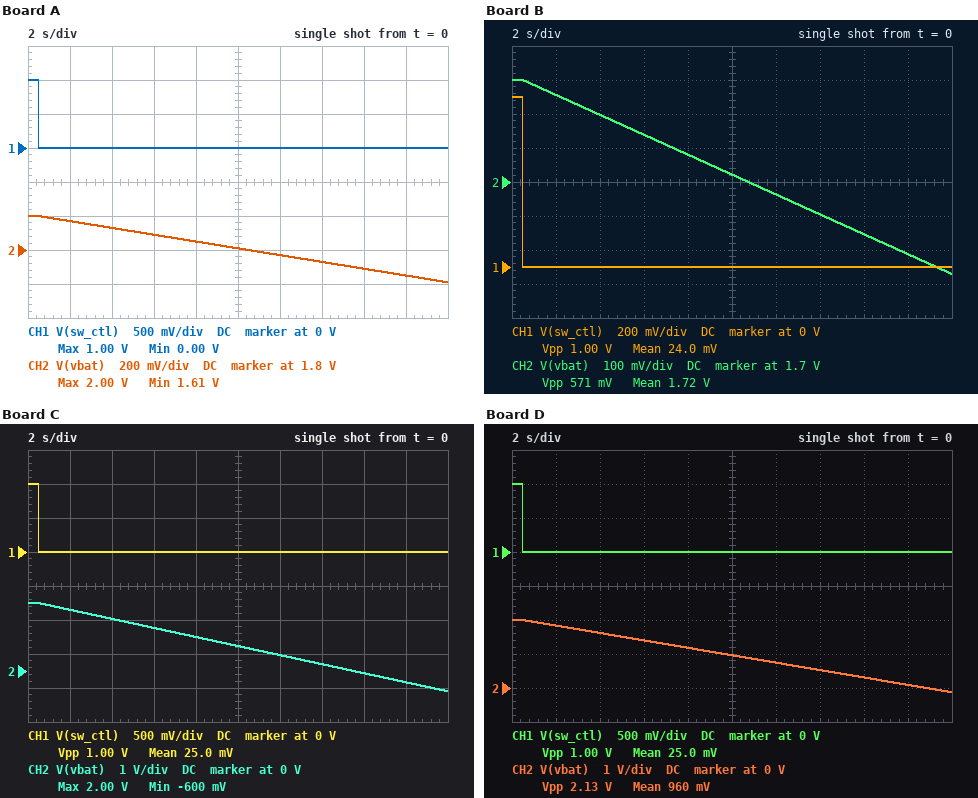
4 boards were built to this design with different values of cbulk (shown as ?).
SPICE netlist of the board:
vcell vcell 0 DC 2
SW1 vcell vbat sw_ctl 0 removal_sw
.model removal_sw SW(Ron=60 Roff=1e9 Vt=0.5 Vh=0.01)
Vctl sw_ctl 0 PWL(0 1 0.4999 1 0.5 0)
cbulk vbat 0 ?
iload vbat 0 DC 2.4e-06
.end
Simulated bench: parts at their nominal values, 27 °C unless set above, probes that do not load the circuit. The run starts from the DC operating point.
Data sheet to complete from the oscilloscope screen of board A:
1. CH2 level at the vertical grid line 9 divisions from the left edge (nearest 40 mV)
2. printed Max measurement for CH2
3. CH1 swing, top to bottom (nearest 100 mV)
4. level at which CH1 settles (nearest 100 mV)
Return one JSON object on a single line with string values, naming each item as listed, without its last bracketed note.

{"CH2 level at the vertical grid line 9 divisions from the left edge": "1.64 V", "printed Max measurement for CH2": "2.00 V", "CH1 swing, top to bottom": "1.0 V", "level at which CH1 settles": "0 V"}
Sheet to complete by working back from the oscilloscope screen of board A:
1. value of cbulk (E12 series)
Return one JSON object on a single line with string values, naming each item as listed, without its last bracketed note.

{"value of cbulk": "120 µF"}
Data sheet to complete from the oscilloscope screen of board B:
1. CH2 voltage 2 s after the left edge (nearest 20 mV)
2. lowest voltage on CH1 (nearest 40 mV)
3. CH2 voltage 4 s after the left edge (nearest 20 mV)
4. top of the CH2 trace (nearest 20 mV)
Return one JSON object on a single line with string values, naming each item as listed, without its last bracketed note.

{"CH2 voltage 2 s after the left edge": "1.96 V", "lowest voltage on CH1": "0 V", "CH2 voltage 4 s after the left edge": "1.90 V", "top of the CH2 trace": "2.00 V"}
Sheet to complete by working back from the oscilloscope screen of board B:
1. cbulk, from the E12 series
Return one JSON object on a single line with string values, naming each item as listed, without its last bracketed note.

{"cbulk, from the E12 series": "82 µF"}
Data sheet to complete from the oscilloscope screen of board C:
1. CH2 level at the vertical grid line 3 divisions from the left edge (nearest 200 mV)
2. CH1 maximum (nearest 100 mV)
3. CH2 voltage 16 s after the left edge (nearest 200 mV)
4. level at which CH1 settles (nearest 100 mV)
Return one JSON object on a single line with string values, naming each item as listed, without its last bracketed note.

{"CH2 level at the vertical grid line 3 divisions from the left edge": "1.2 V", "CH1 maximum": "1.0 V", "CH2 voltage 16 s after the left edge": "0 V", "level at which CH1 settles": "0 V"}
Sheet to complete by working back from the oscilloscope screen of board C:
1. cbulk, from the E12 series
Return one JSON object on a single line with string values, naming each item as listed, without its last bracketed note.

{"cbulk, from the E12 series": "18 µF"}
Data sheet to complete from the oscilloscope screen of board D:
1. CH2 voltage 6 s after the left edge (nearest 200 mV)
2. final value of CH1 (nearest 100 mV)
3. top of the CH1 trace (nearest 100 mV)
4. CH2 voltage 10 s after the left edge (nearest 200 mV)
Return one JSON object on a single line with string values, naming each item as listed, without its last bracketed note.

{"CH2 voltage 6 s after the left edge": "1.4 V", "final value of CH1": "0 V", "top of the CH1 trace": "1.0 V", "CH2 voltage 10 s after the left edge": "1.0 V"}
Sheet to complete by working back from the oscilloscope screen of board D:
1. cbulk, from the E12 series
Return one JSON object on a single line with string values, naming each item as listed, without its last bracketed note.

{"cbulk, from the E12 series": "22 µF"}
